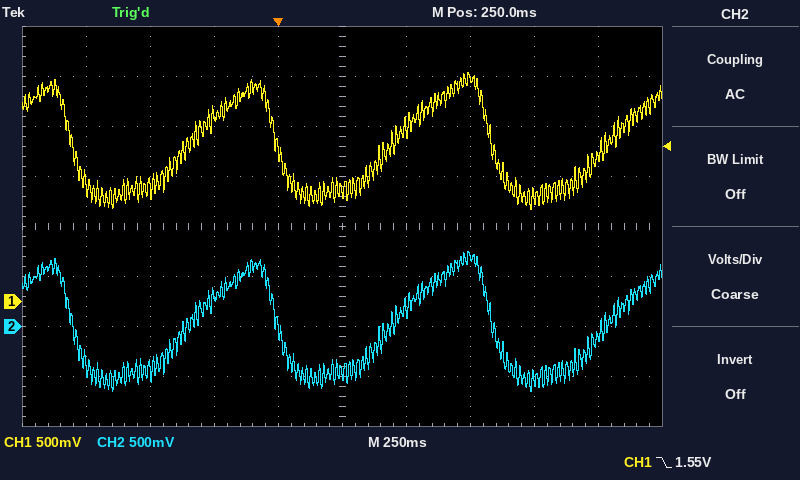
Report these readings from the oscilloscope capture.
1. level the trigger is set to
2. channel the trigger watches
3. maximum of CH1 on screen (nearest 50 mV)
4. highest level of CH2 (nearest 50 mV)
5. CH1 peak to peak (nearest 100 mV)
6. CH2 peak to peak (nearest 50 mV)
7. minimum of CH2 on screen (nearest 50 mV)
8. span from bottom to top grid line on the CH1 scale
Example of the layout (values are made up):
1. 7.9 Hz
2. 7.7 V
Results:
1. 1.55 V
2. CH1
3. 2.30 V
4. 750 mV
5. 1.40 V
6. 1.40 V
7. -650 mV
8. 4 V
